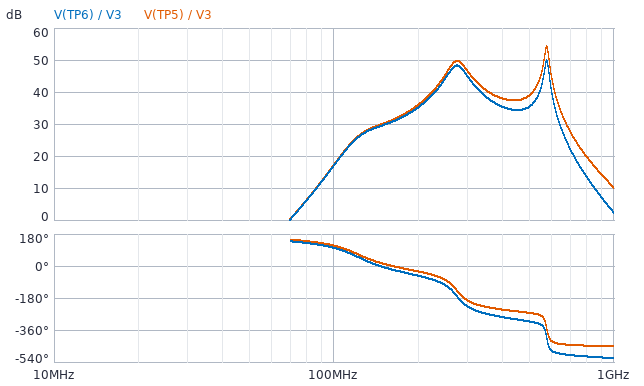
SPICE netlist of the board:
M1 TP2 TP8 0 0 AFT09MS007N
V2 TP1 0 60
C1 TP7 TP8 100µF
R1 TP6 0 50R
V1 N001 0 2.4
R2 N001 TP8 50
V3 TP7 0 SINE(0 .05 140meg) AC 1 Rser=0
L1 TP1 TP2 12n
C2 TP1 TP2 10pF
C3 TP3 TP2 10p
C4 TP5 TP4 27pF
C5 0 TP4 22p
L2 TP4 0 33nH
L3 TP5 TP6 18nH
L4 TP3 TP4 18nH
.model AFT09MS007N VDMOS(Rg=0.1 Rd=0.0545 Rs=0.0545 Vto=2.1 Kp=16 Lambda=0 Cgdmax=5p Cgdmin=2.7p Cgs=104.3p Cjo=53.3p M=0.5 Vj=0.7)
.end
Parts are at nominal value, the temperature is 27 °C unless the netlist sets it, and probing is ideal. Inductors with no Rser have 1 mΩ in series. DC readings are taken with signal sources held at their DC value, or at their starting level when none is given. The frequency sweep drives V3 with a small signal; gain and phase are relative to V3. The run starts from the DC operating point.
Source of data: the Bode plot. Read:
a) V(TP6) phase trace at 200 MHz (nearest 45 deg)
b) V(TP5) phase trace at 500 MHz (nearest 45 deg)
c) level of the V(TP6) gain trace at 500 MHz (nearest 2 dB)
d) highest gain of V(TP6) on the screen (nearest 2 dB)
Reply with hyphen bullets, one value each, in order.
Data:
- -45 deg
- -270 deg
- 36 dB
- 50 dB
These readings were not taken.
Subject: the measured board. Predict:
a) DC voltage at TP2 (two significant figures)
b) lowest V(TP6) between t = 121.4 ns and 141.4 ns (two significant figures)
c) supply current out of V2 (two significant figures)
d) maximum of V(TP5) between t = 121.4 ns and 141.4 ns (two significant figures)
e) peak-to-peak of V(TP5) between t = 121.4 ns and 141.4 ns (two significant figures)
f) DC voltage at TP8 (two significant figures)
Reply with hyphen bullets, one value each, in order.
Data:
- 60 V
- -1.8 V
- 600 mA
- 1.2 V
- 3.2 V
- 2.4 V
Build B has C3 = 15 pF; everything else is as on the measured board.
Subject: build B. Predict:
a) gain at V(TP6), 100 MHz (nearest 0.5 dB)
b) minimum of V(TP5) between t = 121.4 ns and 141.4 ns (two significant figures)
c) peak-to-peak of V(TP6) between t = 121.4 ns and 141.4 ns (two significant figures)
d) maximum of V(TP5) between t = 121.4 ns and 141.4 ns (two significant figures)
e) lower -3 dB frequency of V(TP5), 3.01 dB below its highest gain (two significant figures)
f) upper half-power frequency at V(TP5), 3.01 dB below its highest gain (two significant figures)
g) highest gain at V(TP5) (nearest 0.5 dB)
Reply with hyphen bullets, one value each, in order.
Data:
- 23.0 dB
- -2.4 V
- 3.8 V
- 1.6 V
- 530 MHz
- 550 MHz
- 54.0 dB
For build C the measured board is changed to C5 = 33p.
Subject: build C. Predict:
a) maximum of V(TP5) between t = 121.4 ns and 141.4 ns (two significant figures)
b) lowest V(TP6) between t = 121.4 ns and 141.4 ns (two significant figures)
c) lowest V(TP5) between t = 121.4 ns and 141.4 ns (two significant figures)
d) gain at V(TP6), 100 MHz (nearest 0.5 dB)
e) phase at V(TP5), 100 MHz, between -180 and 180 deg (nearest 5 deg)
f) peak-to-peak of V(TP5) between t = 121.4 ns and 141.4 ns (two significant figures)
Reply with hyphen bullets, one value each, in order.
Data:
- 940 mV
- -1.4 V
- -1.5 V
- 20.0 dB
- 100 deg
- 2.4 V
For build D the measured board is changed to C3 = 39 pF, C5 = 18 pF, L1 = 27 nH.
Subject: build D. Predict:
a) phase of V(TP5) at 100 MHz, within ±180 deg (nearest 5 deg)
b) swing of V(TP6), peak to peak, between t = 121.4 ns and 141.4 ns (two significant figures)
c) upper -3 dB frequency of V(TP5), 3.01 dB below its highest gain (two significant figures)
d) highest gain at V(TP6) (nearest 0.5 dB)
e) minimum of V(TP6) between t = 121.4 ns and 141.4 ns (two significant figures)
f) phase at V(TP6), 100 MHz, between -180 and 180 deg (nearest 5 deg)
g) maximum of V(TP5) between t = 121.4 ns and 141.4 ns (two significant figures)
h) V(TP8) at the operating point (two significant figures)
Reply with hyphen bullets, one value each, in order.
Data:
- -30 deg
- 8.9 V
- 520 MHz
- 45.0 dB
- -4.4 V
- -40 deg
- 4.7 V
- 2.4 V
